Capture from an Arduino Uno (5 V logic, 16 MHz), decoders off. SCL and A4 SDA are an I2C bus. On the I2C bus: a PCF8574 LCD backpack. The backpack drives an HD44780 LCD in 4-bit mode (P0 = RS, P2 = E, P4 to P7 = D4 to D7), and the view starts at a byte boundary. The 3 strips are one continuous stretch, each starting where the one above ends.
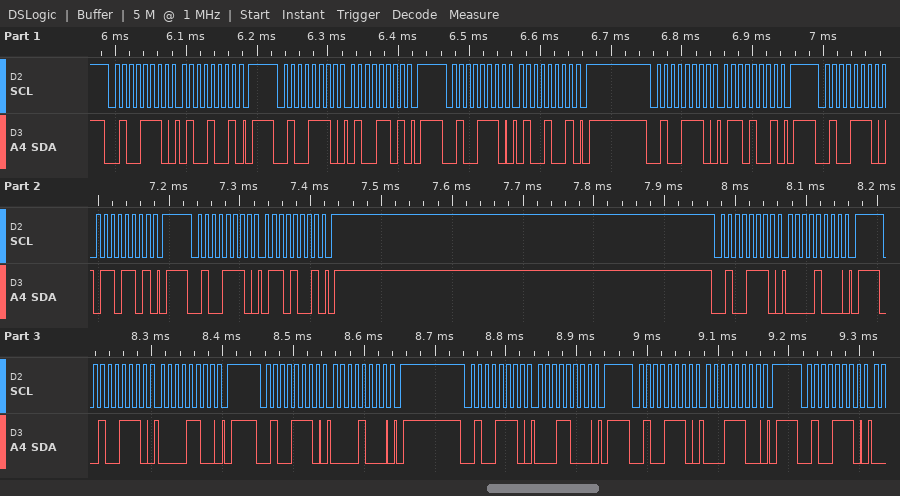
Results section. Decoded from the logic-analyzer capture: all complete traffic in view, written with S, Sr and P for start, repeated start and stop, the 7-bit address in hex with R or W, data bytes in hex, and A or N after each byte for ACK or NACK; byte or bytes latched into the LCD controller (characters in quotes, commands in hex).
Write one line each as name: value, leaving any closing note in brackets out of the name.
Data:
all complete traffic in view, written with S, Sr and P for start, repeated start and stop, the 7-bit address in hex with R or W, data bytes in hex, and A or N after each byte for ACK or NACK: S 27W A 49 A P S 27W A 4D A P S 27W A 49 A P S 27W A 69 A P S 27W A 6D A P S 27W A 69 A P S 27W A 08 A P S 27W A 0C A P S 27W A 08 A P S 27W A 18 A P S 27W A 1C A P S 27W A
byte or bytes latched into the LCD controller: 'F'
